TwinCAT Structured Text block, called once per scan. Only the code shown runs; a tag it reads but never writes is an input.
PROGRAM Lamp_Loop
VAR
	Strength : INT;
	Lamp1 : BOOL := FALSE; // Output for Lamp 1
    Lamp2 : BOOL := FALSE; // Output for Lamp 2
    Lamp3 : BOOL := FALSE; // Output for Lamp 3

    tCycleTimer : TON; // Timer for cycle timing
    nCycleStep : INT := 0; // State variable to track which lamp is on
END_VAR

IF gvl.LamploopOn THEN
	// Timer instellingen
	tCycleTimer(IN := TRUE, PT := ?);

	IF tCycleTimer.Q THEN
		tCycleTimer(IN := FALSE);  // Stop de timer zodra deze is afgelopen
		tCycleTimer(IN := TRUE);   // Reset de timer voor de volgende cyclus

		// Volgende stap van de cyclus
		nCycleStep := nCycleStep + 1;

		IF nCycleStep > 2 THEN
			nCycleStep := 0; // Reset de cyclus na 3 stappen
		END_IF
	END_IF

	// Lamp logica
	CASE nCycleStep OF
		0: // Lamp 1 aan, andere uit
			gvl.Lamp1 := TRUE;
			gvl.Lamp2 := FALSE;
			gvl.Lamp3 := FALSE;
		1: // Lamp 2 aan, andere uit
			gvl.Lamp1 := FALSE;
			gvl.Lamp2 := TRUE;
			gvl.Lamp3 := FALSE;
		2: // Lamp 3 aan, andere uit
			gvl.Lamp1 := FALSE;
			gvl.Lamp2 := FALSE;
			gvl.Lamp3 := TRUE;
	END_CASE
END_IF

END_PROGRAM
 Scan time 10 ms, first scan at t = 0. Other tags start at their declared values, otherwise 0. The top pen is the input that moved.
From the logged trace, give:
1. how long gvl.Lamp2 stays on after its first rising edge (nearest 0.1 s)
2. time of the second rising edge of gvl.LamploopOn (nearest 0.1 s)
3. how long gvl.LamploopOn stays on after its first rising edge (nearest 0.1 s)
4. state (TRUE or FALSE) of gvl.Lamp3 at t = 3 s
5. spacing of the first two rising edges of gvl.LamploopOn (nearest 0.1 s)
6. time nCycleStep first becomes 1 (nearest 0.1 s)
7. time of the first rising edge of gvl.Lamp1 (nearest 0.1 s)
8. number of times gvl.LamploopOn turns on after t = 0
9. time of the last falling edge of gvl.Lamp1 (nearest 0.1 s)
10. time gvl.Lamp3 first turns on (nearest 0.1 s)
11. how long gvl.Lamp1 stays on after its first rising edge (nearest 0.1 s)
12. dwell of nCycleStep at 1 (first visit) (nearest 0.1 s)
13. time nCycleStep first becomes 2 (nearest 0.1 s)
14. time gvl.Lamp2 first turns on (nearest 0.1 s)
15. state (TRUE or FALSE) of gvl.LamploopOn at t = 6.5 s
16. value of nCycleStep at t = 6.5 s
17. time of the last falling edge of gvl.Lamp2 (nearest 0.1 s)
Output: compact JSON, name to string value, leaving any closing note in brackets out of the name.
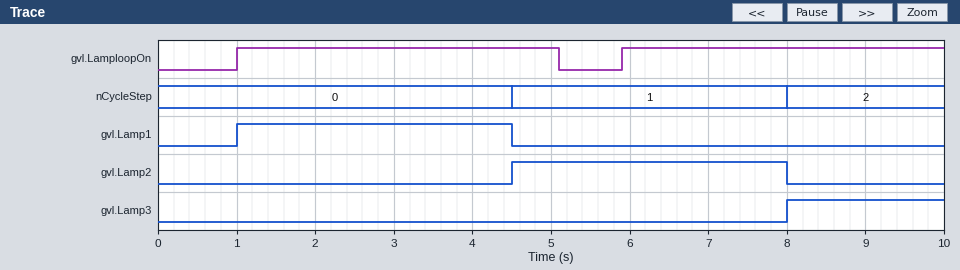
{"how long gvl.Lamp2 stays on after its first rising edge": "3.5 s", "time of the second rising edge of gvl.LamploopOn": "5.9 s", "how long gvl.LamploopOn stays on after its first rising edge": "4.1 s", "state (TRUE or FALSE) of gvl.Lamp3 at t = 3 s": "FALSE", "spacing of the first two rising edges of gvl.LamploopOn": "4.9 s", "time nCycleStep first becomes 1": "4.5 s", "time of the first rising edge of gvl.Lamp1": "1.0 s", "number of times gvl.LamploopOn turns on after t = 0": "2", "time of the last falling edge of gvl.Lamp1": "4.5 s", "time gvl.Lamp3 first turns on": "8.0 s", "how long gvl.Lamp1 stays on after its first rising edge": "3.5 s", "dwell of nCycleStep at 1 (first visit)": "3.5 s", "time nCycleStep first becomes 2": "8.0 s", "time gvl.Lamp2 first turns on": "4.5 s", "state (TRUE or FALSE) of gvl.LamploopOn at t = 6.5 s": "TRUE", "value of nCycleStep at t = 6.5 s": "1", "time of the last falling edge of gvl.Lamp2": "8.0 s"}
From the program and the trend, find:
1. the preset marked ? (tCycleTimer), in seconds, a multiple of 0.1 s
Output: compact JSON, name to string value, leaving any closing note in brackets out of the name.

{"the preset marked ? (tCycleTimer), in seconds, a multiple of 0.1 s": "3.5 s"}
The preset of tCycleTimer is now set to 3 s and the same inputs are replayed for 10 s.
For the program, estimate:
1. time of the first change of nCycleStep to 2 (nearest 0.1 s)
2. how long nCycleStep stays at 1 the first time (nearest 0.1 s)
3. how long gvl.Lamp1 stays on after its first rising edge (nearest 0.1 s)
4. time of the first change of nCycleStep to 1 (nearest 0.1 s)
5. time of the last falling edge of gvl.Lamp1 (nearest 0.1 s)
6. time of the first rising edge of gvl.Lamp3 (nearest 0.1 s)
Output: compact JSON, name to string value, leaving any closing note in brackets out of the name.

{"time of the first change of nCycleStep to 2": "7.0 s", "how long nCycleStep stays at 1 the first time": "3.0 s", "how long gvl.Lamp1 stays on after its first rising edge": "3.0 s", "time of the first change of nCycleStep to 1": "4.0 s", "time of the last falling edge of gvl.Lamp1": "4.0 s", "time of the first rising edge of gvl.Lamp3": "7.0 s"}
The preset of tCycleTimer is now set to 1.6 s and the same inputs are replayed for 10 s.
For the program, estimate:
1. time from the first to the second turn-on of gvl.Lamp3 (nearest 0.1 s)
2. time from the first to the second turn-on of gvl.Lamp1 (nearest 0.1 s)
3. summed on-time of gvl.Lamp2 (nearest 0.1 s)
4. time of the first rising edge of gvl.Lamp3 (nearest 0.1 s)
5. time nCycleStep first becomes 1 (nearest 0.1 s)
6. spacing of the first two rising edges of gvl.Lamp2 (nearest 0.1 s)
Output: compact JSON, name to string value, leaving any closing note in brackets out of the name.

{"time from the first to the second turn-on of gvl.Lamp3": "4.9 s", "time from the first to the second turn-on of gvl.Lamp1": "4.9 s", "summed on-time of gvl.Lamp2": "3.2 s", "time of the first rising edge of gvl.Lamp3": "4.2 s", "time nCycleStep first becomes 1": "2.6 s", "spacing of the first two rising edges of gvl.Lamp2": "4.9 s"}
